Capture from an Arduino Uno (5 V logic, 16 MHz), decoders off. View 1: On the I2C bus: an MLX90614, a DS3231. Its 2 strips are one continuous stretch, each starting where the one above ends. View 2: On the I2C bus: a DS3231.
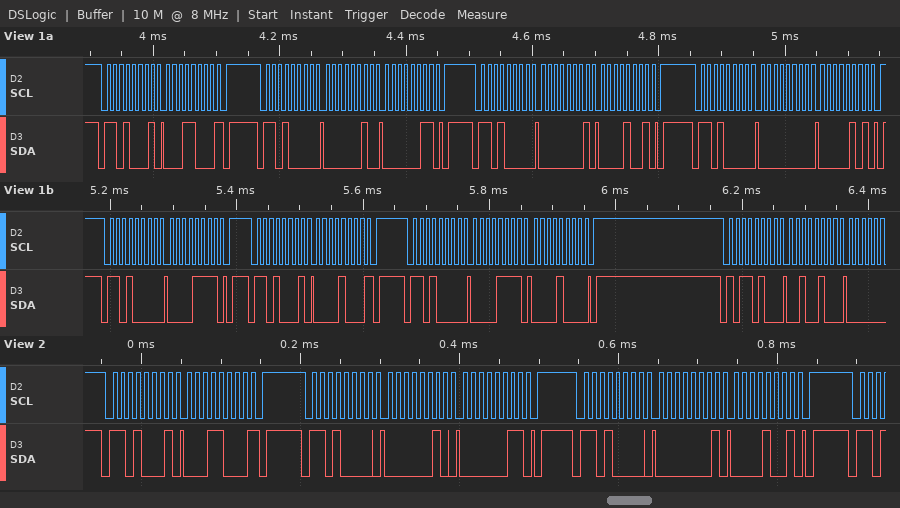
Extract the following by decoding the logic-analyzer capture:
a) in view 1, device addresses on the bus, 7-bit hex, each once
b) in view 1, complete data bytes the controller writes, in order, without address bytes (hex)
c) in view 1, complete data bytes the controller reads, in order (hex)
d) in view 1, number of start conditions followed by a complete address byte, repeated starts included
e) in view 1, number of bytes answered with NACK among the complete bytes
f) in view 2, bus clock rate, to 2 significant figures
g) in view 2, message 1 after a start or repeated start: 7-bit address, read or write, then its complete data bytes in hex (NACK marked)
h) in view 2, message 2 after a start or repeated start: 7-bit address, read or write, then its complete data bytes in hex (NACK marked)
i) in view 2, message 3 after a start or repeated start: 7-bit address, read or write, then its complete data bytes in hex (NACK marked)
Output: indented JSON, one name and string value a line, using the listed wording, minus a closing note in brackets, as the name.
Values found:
{
  "in view 1, device addresses on the bus, 7-bit hex, each once": "0x68 0x5A",
  "in view 1, complete data bytes the controller writes, in order, without address bytes": "02 03 01 09 00 05 0F 0F 08 24",
  "in view 1, complete data bytes the controller reads, in order": "18 08",
  "in view 1, number of start conditions followed by a complete address byte, repeated starts included": "8",
  "in view 1, number of bytes answered with NACK among the complete bytes": "2",
  "in view 2, bus clock rate, to 2 significant figures": "100 kHz",
  "in view 2, message 1 after a start or repeated start: 7-bit address, read or write, then its complete data bytes in hex": "0x68 read: 18 NACK",
  "in view 2, message 2 after a start or repeated start: 7-bit address, read or write, then its complete data bytes in hex": "0x68 write: 02 03",
  "in view 2, message 3 after a start or repeated start: 7-bit address, read or write, then its complete data bytes in hex": "0x68 write: 01 09"
}
